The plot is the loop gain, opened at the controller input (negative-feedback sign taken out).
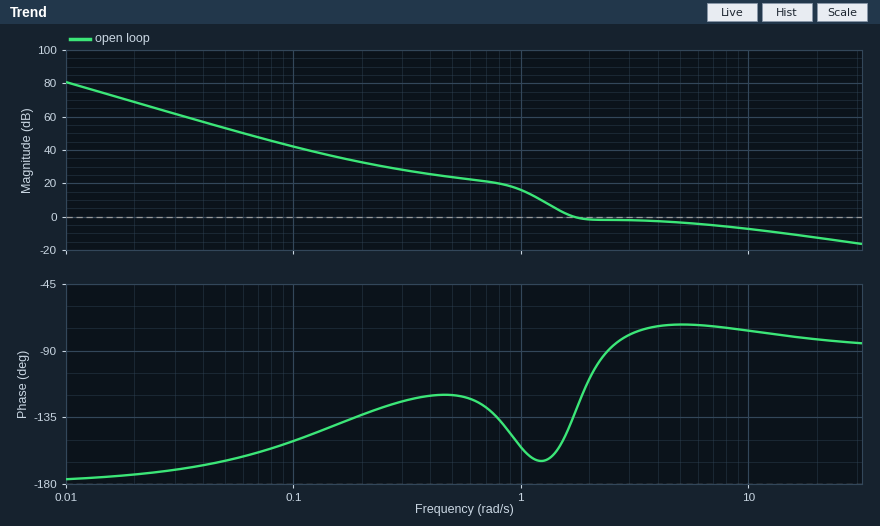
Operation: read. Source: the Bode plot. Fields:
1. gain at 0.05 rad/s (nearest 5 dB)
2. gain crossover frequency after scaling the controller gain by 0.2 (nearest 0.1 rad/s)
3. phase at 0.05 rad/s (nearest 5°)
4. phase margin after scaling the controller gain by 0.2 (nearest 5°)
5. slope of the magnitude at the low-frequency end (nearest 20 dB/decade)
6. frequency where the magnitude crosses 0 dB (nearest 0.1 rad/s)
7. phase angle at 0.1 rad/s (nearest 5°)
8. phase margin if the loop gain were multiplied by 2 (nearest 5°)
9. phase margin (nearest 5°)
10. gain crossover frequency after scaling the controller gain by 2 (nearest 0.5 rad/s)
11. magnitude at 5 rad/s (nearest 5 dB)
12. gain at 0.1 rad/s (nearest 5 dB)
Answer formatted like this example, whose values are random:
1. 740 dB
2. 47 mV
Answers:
1. 55 dB
2. 1.1 rad/s
3. -165°
4. 20°
5. -40 dB/decade
6. 1.7 rad/s
7. -150°
8. 105°
9. 45°
10. 8.0 rad/s
11. -5 dB
12. 40 dB
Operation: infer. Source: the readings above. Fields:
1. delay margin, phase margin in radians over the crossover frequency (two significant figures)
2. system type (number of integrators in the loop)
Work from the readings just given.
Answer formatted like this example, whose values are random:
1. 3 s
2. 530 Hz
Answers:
1. 0.46 s
2. 2
